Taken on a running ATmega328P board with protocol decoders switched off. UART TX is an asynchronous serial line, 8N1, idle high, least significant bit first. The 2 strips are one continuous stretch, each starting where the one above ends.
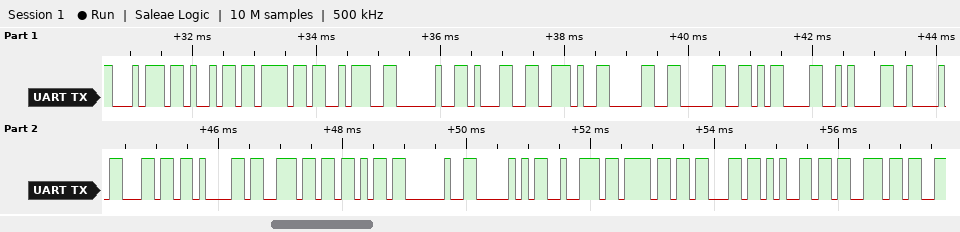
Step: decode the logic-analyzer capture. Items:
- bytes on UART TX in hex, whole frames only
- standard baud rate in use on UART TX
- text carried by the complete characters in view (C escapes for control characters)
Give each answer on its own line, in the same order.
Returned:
74 69 6F 3A 20 31 2E 30 30 0D 0A 42 6C 61 6E 6B 20 50 72 6F 63 65 73
9600 baud
"tio: 1.00\r\nBlank Proces"
